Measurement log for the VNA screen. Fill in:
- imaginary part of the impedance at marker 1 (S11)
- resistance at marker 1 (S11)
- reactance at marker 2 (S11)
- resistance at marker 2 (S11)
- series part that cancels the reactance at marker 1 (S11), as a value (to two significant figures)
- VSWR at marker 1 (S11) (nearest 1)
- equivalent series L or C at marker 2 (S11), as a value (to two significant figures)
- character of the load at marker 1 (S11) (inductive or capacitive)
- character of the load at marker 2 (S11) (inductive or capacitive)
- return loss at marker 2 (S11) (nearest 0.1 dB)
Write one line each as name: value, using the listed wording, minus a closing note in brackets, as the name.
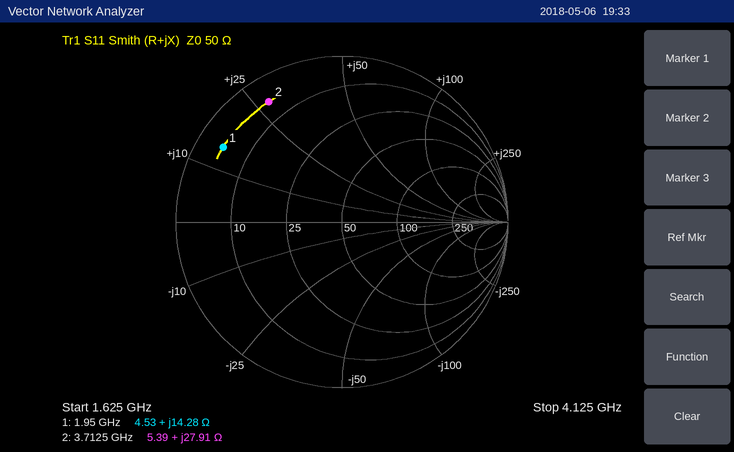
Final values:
imaginary part of the impedance at marker 1: +14.28 Ω
resistance at marker 1: 4.53 Ω
reactance at marker 2: +27.91 Ω
resistance at marker 2: 5.39 Ω
series part that cancels the reactance at marker 1 (S11), as a value: 5.7 pF
VSWR at marker 1 (S11): 12
equivalent series L or C at marker 2 (S11), as a value: 1.2 nH
character of the load at marker 1 (S11): inductive
character of the load at marker 2 (S11): inductive
return loss at marker 2 (S11): 1.4 dB
